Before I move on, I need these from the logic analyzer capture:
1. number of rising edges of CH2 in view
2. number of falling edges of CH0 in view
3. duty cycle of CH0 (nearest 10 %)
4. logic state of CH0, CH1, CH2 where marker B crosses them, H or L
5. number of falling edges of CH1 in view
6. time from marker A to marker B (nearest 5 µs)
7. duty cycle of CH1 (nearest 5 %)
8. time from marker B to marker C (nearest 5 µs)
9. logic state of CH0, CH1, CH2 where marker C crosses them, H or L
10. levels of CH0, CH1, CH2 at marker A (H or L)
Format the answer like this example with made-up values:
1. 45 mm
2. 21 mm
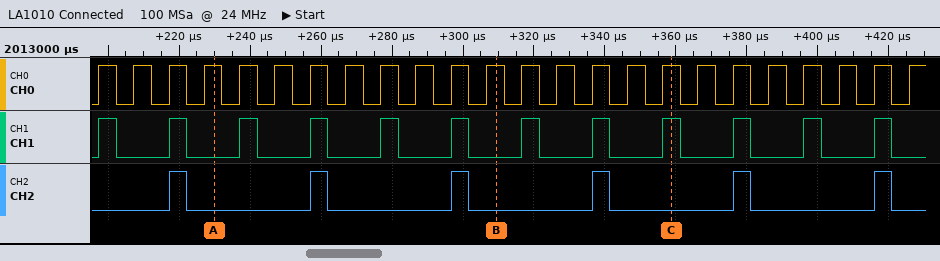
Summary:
1. 6
2. 23
3. 50 %
4. CH0=H, CH1=L, CH2=L
5. 12
6. 80 µs
7. 25 %
8. 50 µs
9. CH0=H, CH1=H, CH2=L
10. CH0=H, CH1=L, CH2=L
